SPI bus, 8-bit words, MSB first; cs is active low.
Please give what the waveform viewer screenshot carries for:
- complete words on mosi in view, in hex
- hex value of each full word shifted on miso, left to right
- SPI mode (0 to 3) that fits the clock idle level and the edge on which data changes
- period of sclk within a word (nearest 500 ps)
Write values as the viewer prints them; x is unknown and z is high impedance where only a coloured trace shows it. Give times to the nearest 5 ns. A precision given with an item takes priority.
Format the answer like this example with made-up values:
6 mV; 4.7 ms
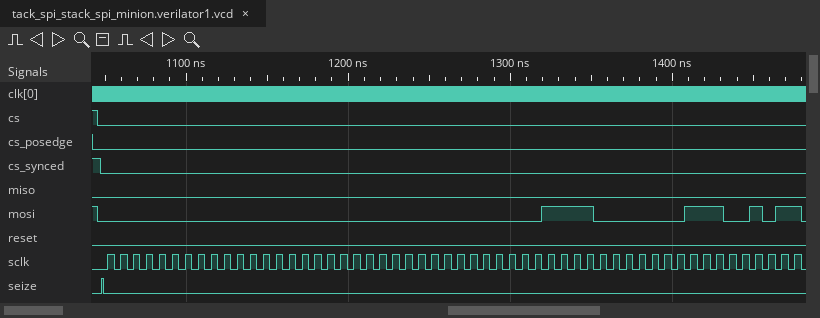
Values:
00, 00, 00, 00, 3C, 07; 00, 00, 00, 00, 00, 00; 0; 8000 ps
